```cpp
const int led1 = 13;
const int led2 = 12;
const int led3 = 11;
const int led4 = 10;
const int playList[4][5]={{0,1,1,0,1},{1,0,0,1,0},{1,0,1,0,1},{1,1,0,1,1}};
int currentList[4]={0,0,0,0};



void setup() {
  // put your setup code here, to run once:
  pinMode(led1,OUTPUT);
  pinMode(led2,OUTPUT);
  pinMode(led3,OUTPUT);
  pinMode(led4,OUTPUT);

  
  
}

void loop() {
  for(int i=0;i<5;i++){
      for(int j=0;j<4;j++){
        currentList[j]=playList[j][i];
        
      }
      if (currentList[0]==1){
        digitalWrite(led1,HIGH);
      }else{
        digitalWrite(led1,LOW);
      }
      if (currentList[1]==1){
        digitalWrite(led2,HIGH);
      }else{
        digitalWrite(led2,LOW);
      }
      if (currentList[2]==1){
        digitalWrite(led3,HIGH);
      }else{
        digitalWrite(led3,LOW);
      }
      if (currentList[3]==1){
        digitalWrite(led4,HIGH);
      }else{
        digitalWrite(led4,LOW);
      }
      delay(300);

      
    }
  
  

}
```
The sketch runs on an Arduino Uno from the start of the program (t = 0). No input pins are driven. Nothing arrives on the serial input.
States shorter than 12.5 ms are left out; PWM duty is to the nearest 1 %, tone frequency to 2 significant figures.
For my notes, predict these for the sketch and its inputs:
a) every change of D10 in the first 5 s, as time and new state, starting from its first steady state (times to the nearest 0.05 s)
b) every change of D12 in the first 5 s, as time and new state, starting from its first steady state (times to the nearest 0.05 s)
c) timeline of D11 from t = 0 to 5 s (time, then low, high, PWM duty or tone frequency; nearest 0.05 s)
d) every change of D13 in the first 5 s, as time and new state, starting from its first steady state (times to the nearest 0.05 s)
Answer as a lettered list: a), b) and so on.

a) 0 s high; 0.6 s low; 0.9 s high; 2.1 s low; 2.4 s high; 3.6 s low; 3.9 s high
b) 0 s high; 0.3 s low; 0.9 s high; 1.2 s low; 1.5 s high; 1.8 s low; 2.4 s high; 2.7 s low; 3 s high; 3.3 s low; 3.9 s high; 4.2 s low; 4.5 s high; 4.8 s low
c) 0 s high; 0.3 s low; 0.6 s high; 0.9 s low; 1.2 s high; 1.8 s low; 2.1 s high; 2.4 s low; 2.7 s high; 3.3 s low; 3.6 s high; 3.9 s low; 4.2 s high; 4.8 s low
d) 0 s low; 0.3 s high; 0.9 s low; 1.2 s high; 1.5 s low; 1.8 s high; 2.4 s low; 2.7 s high; 3 s low; 3.3 s high; 3.9 s low; 4.2 s high; 4.5 s low; 4.8 s high
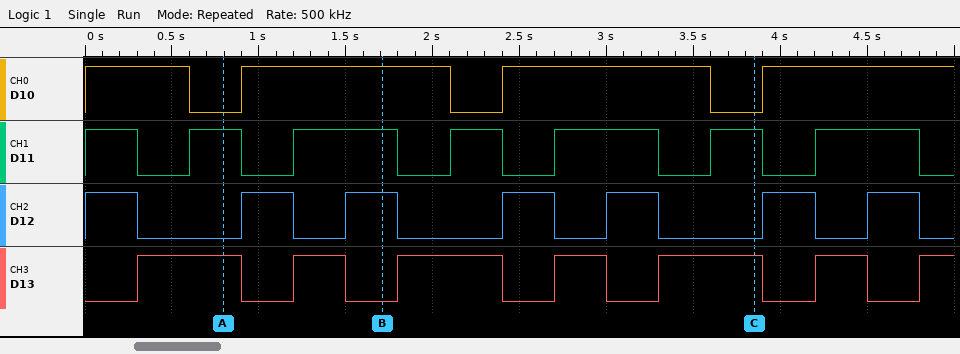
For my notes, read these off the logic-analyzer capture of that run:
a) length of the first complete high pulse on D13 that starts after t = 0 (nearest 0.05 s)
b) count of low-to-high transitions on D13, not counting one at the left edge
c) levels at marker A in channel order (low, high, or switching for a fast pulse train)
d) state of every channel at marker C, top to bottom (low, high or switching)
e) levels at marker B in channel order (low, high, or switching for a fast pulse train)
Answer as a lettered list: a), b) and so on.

a) 0.60 s
b) 7
c) D10 low, D11 high, D12 low, D13 high
d) D10 low, D11 high, D12 low, D13 high
e) D10 high, D11 high, D12 high, D13 low
